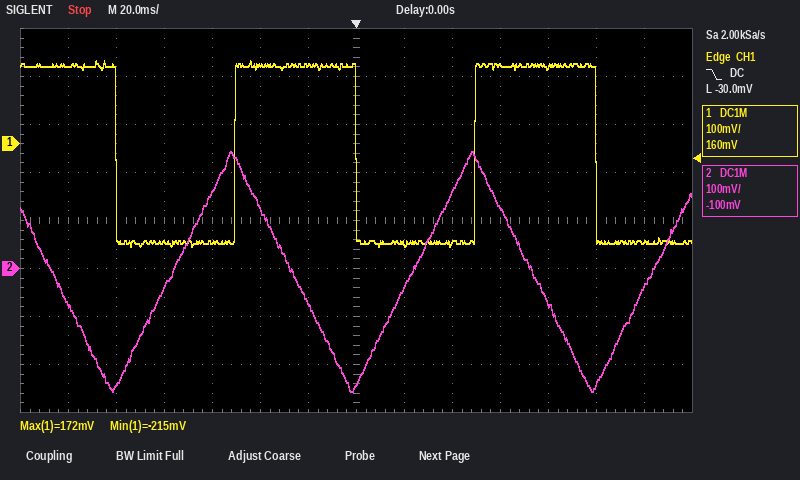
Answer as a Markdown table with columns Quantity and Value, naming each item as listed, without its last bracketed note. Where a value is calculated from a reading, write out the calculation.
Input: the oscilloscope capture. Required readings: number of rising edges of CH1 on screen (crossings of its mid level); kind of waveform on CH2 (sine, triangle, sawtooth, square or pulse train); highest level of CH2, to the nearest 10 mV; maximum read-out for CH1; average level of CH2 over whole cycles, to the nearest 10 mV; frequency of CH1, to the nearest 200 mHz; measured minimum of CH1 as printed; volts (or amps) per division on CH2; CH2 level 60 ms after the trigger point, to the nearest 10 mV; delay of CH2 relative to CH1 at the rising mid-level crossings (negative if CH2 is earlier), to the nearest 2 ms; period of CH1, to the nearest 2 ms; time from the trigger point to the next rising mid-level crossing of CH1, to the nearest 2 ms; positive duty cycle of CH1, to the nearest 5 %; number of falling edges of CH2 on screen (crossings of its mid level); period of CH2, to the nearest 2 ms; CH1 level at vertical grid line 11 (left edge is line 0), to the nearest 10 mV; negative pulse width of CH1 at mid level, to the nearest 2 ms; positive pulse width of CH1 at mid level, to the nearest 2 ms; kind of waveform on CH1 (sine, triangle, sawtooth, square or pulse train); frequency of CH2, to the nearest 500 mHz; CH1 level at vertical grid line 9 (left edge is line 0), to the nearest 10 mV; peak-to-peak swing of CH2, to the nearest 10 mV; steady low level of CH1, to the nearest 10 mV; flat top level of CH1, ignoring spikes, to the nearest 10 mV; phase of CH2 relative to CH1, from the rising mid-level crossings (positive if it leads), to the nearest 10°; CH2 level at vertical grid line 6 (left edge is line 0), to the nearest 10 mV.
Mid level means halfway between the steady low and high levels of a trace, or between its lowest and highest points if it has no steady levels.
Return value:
| Quantity | Value |
|---|---|
| number of rising edges of CH1 on screen | 2 |
| kind of waveform on CH2 | triangle |
| highest level of CH2, to the nearest 10 mV | 240 mV |
| maximum read-out for CH1 | 172 mV |
| average level of CH2 over whole cycles, to the nearest 10 mV | (240 mV + (-260 mV)) / 2 ≈ -10 mV |
| frequency of CH1, to the nearest 200 mHz | 1 / 100 ms ≈ 10.0 Hz |
| measured minimum of CH1 as printed | -215 mV |
| volts (or amps) per division on CH2 | 100 mV |
| CH2 level 60 ms after the trigger point, to the nearest 10 mV | 130 mV |
| delay of CH2 relative to CH1 at the rising mid-level crossings (negative if CH2 is earlier), to the nearest 2 ms | -26 ms |
| period of CH1, to the nearest 2 ms | 100 ms |
| time from the trigger point to the next rising mid-level crossing of CH1, to the nearest 2 ms | 50 ms |
| positive duty cycle of CH1, to the nearest 5 % | 50 ms / 100 ms ≈ 50 % |
| number of falling edges of CH2 on screen | 3 |
| period of CH2, to the nearest 2 ms | 100 ms |
| CH1 level at vertical grid line 11 (left edge is line 0), to the nearest 10 mV | 160 mV |
| negative pulse width of CH1 at mid level, to the nearest 2 ms | 50 ms |
| positive pulse width of CH1 at mid level, to the nearest 2 ms | 50 ms |
| kind of waveform on CH1 | square |
| frequency of CH2, to the nearest 500 mHz | 1 / 100 ms ≈ 10.0 Hz |
| CH1 level at vertical grid line 9 (left edge is line 0), to the nearest 10 mV | -210 mV |
| peak-to-peak swing of CH2, to the nearest 10 mV | 240 mV − (-260 mV) = 500 mV |
| steady low level of CH1, to the nearest 10 mV | -210 mV |
| flat top level of CH1, ignoring spikes, to the nearest 10 mV | 160 mV |
| phase of CH2 relative to CH1, from the rising mid-level crossings (positive if it leads), to the nearest 10° | −360° × (-26 ms) / 100 ms ≈ +93.6°, so +90° to the nearest 10° |
| CH2 level at vertical grid line 6 (left edge is line 0), to the nearest 10 mV | -70 mV |
